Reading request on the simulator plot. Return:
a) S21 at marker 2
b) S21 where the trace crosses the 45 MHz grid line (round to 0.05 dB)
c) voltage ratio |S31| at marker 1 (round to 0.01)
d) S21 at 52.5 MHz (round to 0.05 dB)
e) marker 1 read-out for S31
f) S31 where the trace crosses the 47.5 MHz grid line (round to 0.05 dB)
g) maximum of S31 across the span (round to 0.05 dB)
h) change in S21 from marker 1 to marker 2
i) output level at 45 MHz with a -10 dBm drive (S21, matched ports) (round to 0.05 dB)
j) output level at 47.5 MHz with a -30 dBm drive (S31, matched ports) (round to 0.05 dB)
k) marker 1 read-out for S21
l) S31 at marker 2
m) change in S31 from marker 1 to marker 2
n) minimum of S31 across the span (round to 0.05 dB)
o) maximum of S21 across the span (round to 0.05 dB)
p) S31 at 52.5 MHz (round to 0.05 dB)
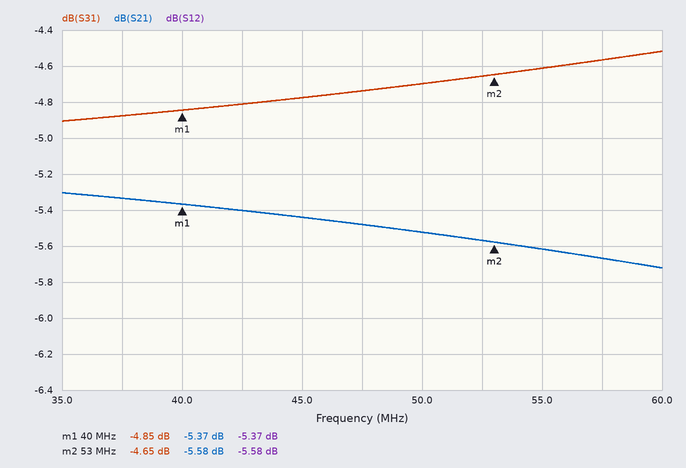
-5.58 dB
-5.45 dB
0.57
-5.55 dB
-4.85 dB
-4.75 dB
-4.50 dB
-0.21 dB
-15.45 dBm
-34.75 dBm
-5.37 dB
-4.65 dB
0.20 dB
-4.90 dB
-5.30 dB
-4.65 dB
